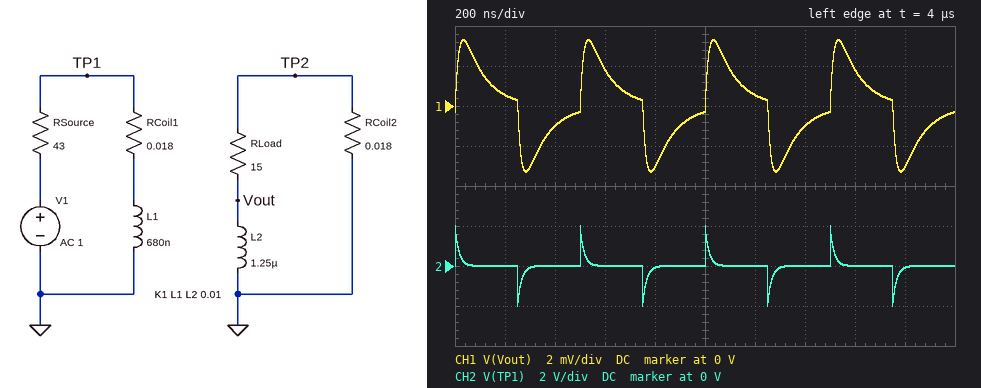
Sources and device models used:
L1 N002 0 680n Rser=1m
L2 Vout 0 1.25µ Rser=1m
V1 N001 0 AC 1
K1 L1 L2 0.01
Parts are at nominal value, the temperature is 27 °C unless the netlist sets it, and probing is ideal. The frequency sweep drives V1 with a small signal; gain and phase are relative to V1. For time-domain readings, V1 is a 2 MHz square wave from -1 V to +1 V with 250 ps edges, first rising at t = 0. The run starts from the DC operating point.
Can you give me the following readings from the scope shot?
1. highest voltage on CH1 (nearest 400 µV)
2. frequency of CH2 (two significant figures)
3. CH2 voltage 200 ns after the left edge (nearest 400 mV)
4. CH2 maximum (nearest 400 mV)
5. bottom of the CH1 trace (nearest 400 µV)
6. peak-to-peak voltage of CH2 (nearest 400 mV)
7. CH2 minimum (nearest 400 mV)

3.2 mV
2.0 MHz
0 V
2.0 V
-3.2 mV
4.0 V
-2.0 V
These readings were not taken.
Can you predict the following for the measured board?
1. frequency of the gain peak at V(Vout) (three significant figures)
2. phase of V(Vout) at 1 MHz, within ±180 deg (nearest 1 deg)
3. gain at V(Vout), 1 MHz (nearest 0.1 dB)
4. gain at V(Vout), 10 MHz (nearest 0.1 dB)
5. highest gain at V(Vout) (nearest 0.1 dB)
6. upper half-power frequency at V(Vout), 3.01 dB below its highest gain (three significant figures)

4.39 MHz
57 deg
-58.5 dB
-54.9 dB
-53.3 dB
13.4 MHz
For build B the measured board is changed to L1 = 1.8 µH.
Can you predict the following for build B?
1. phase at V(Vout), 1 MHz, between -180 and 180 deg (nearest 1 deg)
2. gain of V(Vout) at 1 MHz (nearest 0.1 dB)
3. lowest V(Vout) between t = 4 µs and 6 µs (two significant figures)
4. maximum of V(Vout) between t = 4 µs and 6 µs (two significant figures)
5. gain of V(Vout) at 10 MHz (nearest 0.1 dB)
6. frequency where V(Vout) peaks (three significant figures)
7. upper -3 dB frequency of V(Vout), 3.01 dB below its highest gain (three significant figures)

48 deg
-54.5 dB
-3.8 mV
3.8 mV
-56.7 dB
2.70 MHz
6.79 MHz
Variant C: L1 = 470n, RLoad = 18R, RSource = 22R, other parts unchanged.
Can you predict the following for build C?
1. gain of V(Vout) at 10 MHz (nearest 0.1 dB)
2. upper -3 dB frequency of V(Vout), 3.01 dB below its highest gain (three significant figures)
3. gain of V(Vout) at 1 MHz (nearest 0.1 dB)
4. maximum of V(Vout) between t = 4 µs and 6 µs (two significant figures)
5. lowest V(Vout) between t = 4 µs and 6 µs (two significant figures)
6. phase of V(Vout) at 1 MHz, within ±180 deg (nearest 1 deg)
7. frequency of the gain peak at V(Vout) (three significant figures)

-50.7 dB
11.3 MHz
-54.0 dB
5.7 mV
-5.7 mV
59 deg
4.14 MHz
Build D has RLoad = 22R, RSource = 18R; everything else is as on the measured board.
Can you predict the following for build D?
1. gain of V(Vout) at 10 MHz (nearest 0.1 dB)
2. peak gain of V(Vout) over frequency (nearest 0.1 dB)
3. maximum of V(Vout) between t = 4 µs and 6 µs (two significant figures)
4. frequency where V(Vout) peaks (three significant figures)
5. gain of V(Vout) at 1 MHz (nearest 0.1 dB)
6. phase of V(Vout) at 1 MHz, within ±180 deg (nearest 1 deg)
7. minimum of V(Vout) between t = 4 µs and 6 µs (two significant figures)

-49.4 dB
-45.3 dB
7.8 mV
3.44 MHz
-50.6 dB
57 deg
-7.8 mV
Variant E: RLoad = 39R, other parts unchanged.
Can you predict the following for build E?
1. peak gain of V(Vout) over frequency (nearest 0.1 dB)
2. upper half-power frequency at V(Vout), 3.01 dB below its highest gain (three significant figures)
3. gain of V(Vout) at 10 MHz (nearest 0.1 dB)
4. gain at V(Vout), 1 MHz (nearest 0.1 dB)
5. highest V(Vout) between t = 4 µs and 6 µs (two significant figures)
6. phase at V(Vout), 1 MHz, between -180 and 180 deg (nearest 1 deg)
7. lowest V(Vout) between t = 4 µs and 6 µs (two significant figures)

-47.0 dB
17.8 MHz
-47.4 dB
-57.6 dB
6.7 mV
73 deg
-6.7 mV
